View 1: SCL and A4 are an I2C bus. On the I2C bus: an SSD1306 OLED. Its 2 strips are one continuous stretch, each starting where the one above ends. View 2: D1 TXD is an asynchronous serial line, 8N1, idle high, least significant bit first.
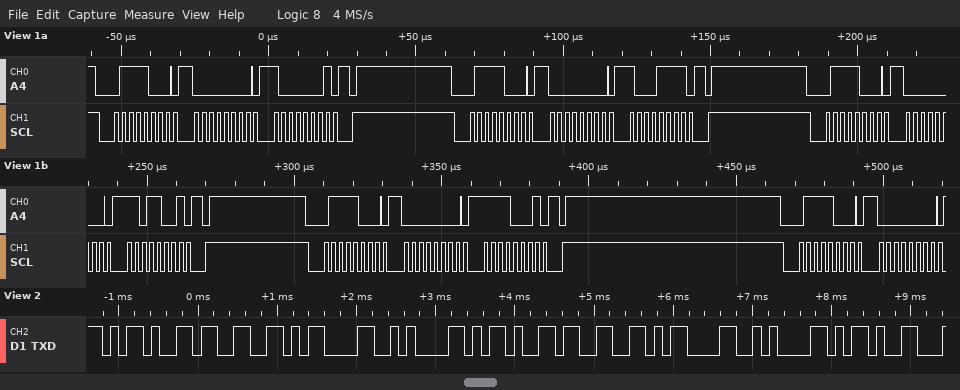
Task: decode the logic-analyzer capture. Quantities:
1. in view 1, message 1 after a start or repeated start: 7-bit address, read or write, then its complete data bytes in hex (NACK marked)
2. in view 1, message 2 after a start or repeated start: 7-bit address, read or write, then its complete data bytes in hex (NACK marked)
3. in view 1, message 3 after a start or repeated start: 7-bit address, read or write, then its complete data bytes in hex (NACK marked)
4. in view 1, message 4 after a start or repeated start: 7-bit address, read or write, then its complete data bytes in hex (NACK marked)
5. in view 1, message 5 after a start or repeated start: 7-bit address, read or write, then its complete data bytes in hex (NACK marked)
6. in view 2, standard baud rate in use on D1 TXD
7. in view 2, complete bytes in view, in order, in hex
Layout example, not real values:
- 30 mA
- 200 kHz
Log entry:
- 0x3C write: 00 81
- 0x3C write: 00 8F
- 0x3C write: 00 D9
- 0x3C write: 00 F1
- 0x3C write: 00
- 9600 baud
- 0x2D 0x33 0x0D 0x0A 0x2D 0x33 0x0D 0x0A 0x2D
